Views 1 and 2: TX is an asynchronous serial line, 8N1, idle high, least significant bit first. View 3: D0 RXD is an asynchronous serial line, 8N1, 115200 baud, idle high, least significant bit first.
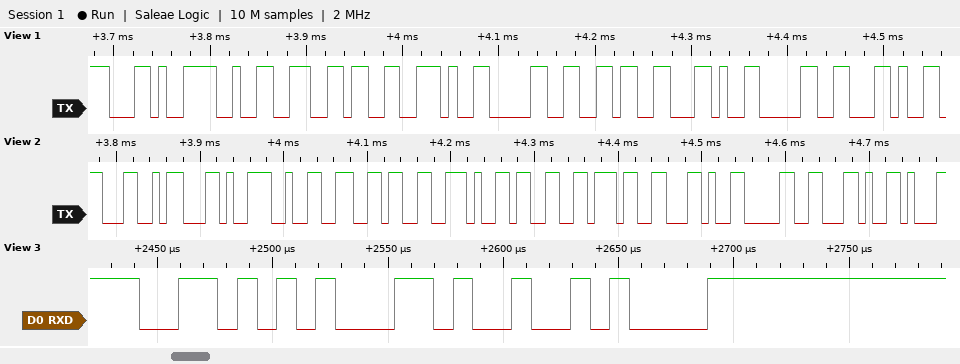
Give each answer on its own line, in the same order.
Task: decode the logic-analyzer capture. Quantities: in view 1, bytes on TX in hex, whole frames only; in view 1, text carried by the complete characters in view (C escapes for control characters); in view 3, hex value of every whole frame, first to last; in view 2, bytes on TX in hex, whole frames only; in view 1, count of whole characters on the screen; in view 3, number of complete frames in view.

0x2C 0x32 0x36 0x2E 0x30 0x36 0x2C 0x30 0x2C
",26.06,0,"
56 2C 0A
4C 2C 32 36 2E 33 37 2C 30 2C
9
3
